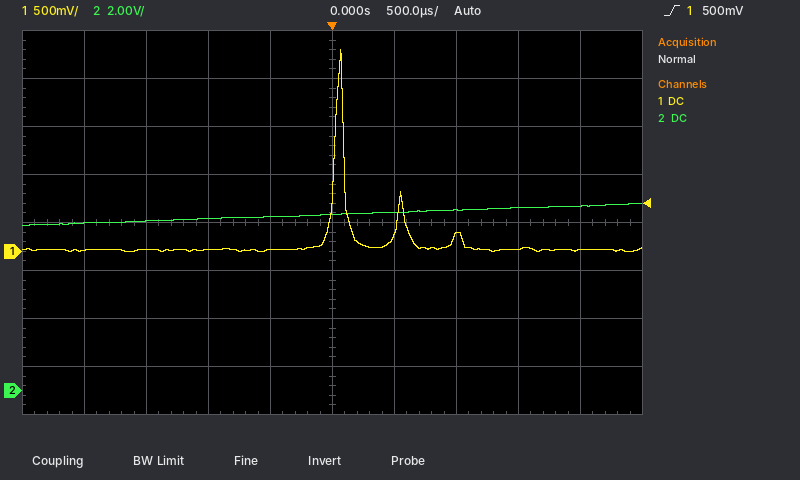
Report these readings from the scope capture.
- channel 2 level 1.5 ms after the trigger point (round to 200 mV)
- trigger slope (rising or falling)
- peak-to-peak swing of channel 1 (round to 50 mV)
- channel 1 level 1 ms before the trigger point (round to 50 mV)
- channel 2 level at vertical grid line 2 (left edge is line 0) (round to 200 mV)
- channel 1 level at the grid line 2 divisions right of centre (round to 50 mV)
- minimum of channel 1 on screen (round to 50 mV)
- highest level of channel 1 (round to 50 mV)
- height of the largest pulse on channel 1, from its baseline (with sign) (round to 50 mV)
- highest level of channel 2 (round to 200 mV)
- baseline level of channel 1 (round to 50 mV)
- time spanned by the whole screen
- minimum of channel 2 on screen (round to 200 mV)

7.6 V
rising
2.10 V
0 mV
7.0 V
150 mV
0 mV
2.10 V
+2.10 V
7.8 V
0 mV
5 ms
6.8 V
